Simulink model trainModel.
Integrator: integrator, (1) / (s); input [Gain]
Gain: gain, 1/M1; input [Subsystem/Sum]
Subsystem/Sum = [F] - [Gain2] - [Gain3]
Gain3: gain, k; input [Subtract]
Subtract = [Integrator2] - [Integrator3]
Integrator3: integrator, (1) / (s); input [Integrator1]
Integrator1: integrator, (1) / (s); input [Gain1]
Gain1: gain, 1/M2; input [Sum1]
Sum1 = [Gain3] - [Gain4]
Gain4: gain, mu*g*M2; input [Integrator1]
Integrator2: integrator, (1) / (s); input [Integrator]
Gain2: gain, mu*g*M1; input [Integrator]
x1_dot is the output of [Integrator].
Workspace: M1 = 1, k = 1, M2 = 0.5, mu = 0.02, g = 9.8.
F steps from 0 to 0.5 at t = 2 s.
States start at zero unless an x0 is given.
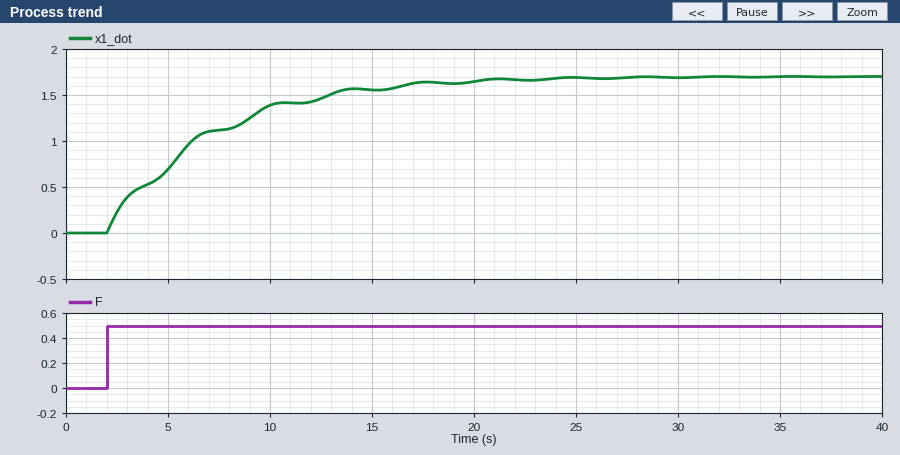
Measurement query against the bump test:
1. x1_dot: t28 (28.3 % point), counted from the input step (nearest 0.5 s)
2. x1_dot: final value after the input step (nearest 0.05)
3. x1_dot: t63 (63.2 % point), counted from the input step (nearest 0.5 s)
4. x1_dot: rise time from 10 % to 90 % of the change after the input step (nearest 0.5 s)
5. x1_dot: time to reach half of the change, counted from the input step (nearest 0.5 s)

1.5 s
1.70
4.5 s
11.0 s
3.5 s
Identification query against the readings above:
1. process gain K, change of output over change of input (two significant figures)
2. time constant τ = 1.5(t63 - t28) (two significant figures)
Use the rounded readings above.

3.4
4.5 s
